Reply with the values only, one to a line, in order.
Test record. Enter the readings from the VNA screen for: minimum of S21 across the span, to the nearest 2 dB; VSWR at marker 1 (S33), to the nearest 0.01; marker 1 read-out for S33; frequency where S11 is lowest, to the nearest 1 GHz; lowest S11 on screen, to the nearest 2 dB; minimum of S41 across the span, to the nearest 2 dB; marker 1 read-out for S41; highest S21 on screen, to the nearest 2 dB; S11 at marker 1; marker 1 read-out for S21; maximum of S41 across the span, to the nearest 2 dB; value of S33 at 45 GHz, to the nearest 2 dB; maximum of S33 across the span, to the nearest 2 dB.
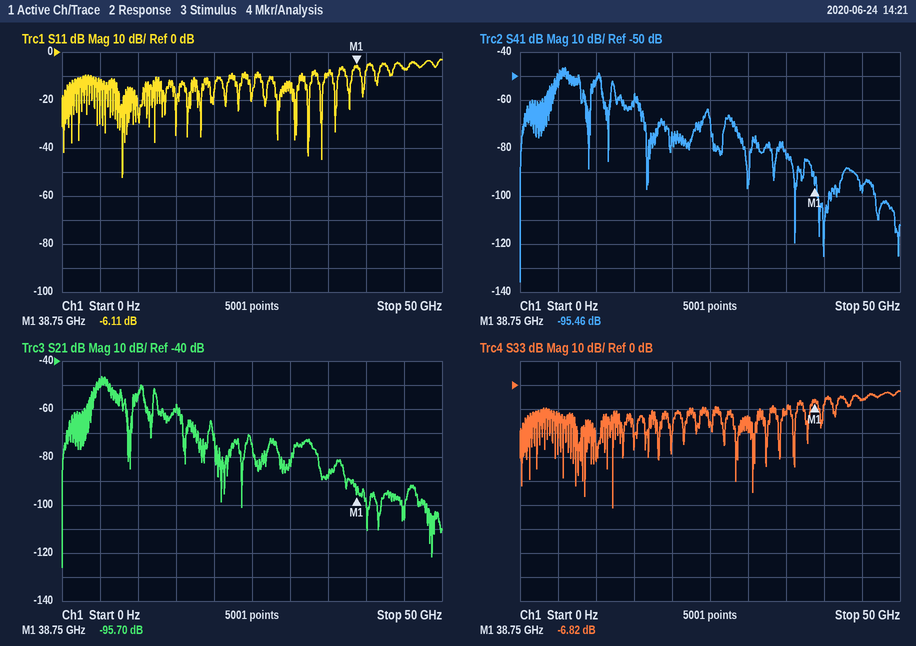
-126 dB
2.68
-6.82 dB
8 GHz
-52 dB
-136 dB
-95.46 dB
-46 dB
-6.11 dB
-95.70 dB
-46 dB
-6 dB
-2 dB
